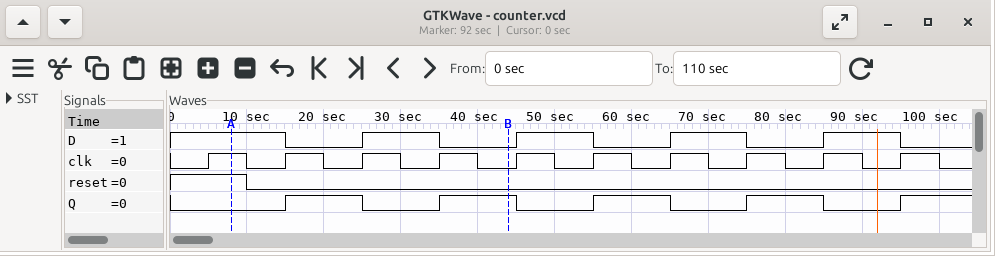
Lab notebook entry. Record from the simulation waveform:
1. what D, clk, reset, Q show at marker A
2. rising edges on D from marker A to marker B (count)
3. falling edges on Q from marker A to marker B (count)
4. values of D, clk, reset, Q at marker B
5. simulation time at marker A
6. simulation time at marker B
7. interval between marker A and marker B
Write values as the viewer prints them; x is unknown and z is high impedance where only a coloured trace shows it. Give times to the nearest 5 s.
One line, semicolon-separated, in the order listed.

D=1, clk=1, reset=1, Q=0; 1; 1; D=0, clk=0, reset=0, Q=1; 10 s; 45 s; 35 s
